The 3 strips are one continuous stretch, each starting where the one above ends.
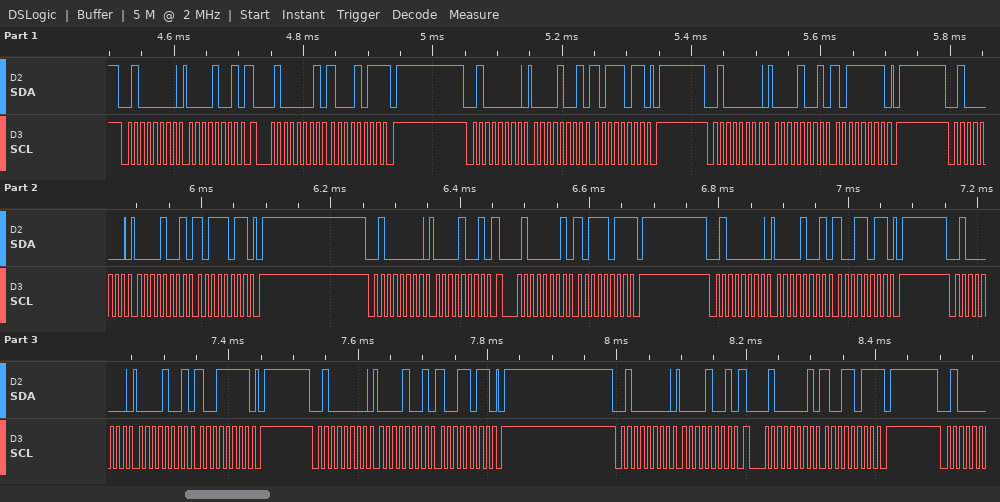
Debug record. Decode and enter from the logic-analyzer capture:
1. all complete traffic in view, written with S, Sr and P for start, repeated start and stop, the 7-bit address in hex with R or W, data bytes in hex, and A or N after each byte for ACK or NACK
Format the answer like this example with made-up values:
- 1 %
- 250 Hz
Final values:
- S 20W A 09 A Sr 20R A 8B N P S 20W A 09 A BB A P S 20W A 09 A BF A P S 20W A 09 A BB A P S 20W A 09 A Sr 20R A BB N P S 20W A 09 A 9B A P S 20W A 09 A 9F A P S 20W A 09 A 9B A P S 20W A 09 A Sr 20R A 9B N P
